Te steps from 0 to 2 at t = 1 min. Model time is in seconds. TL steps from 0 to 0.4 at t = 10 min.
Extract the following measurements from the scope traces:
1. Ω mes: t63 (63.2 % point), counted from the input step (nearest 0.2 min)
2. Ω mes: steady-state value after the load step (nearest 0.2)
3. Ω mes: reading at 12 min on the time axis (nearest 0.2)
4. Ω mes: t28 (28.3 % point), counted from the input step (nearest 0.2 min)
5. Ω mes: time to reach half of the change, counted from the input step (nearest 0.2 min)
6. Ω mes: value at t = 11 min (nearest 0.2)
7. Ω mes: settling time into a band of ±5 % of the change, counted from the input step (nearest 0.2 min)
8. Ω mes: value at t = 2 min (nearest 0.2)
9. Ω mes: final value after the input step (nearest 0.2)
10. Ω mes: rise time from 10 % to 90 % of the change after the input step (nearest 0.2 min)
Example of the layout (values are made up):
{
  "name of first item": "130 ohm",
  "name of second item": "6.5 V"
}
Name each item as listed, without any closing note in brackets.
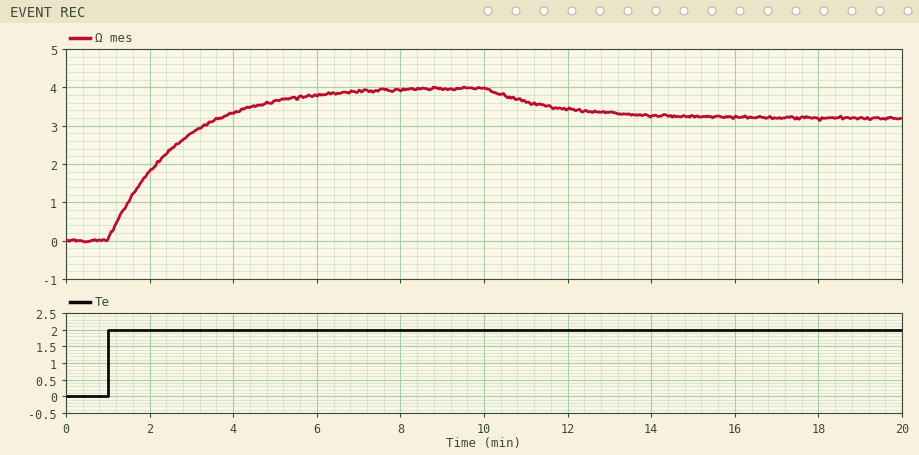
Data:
{
  "Ω mes: t63 (63.2 % point), counted from the input step": "1.6 min",
  "Ω mes: steady-state value after the load step": "3.2",
  "Ω mes: reading at 12 min on the time axis": "3.4",
  "Ω mes: t28 (28.3 % point), counted from the input step": "0.6 min",
  "Ω mes: time to reach half of the change, counted from the input step": "1.2 min",
  "Ω mes: value at t = 11 min": "3.6",
  "Ω mes: settling time into a band of ±5 % of the change, counted from the input step": "5.0 min",
  "Ω mes: value at t = 2 min": "1.8",
  "Ω mes: final value after the input step": "4.0",
  "Ω mes: rise time from 10 % to 90 % of the change after the input step": "3.6 min"
}
